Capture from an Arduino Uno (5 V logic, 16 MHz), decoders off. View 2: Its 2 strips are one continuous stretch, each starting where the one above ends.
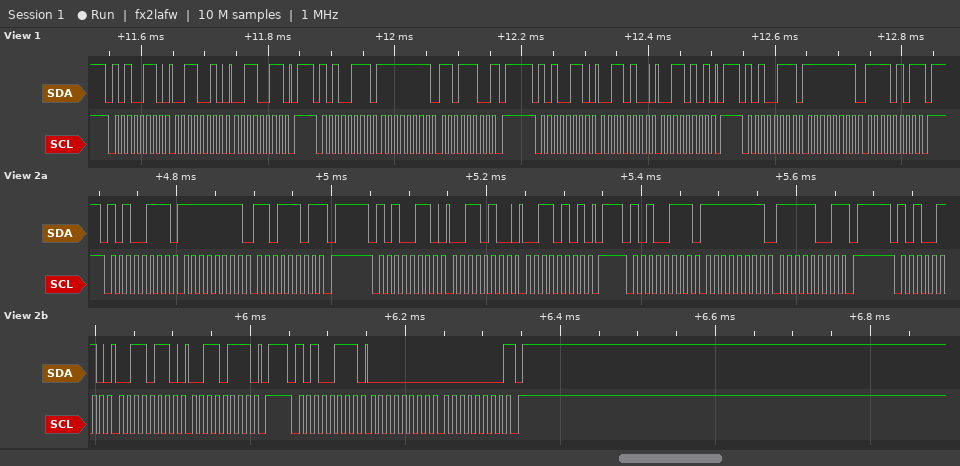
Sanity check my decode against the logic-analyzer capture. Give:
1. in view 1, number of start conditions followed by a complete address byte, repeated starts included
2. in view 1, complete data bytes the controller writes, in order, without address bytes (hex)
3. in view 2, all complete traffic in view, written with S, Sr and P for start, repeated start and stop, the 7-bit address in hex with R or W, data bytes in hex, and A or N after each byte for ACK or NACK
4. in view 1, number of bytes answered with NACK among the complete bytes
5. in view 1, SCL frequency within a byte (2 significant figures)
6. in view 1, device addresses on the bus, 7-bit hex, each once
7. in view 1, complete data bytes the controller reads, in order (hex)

4
32 33 34 35
S 53R A FF A DD N P S 53W A 34 A 35 A P S 53R A FF A F9 N P S 53W A 36 A 37 A P S 53R A 00 A 00 N P
2
100 kHz
0x53
FF DC FF F5
